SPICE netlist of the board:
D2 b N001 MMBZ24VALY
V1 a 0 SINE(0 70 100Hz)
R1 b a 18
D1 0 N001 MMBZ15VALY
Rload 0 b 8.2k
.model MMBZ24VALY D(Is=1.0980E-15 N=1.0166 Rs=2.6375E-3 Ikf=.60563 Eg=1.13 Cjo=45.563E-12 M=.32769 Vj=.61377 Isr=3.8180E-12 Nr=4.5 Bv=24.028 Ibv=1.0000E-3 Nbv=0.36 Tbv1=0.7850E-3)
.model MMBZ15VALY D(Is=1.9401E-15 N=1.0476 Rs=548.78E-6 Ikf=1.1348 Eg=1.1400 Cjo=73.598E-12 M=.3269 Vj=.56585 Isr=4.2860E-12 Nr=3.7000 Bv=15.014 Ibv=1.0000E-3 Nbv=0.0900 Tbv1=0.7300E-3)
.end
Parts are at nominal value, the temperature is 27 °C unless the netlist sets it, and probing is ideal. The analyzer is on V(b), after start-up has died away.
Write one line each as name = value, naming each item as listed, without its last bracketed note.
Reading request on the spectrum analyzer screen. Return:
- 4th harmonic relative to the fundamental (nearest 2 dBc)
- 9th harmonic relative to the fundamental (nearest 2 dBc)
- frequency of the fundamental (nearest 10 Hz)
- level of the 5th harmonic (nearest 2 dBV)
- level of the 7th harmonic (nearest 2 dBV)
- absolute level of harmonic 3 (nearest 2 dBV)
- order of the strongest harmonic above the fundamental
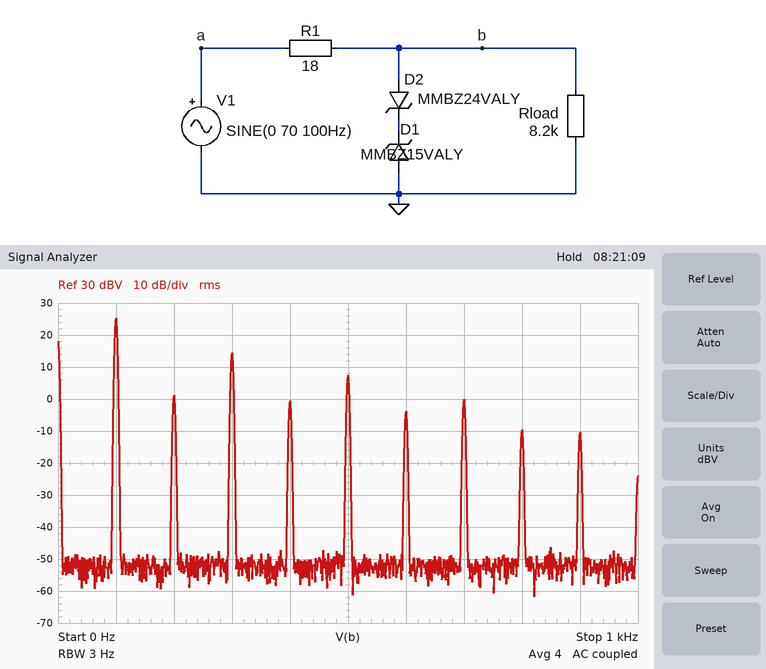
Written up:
4th harmonic relative to the fundamental = -26 dBc
9th harmonic relative to the fundamental = -36 dBc
frequency of the fundamental = 100 Hz
level of the 5th harmonic = 8 dBV
level of the 7th harmonic = 0 dBV
absolute level of harmonic 3 = 14 dBV
order of the strongest harmonic above the fundamental = 3
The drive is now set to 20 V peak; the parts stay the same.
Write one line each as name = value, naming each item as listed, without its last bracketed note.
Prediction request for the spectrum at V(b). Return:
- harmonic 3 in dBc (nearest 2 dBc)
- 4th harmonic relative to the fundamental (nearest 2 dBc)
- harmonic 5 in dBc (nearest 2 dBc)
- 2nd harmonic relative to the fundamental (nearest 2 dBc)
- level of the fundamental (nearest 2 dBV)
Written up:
harmonic 3 in dBc = -28 dBc
4th harmonic relative to the fundamental = -32 dBc
harmonic 5 in dBc = -36 dBc
2nd harmonic relative to the fundamental = -26 dBc
level of the fundamental = 22 dBV
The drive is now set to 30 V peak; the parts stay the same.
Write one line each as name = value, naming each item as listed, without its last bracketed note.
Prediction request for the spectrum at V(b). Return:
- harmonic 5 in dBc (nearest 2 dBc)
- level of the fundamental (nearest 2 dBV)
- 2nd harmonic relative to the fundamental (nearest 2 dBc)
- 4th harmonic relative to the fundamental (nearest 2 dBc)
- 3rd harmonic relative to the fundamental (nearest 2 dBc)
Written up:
harmonic 5 in dBc = -44 dBc
level of the fundamental = 24 dBV
2nd harmonic relative to the fundamental = -18 dBc
4th harmonic relative to the fundamental = -44 dBc
3rd harmonic relative to the fundamental = -18 dBc
